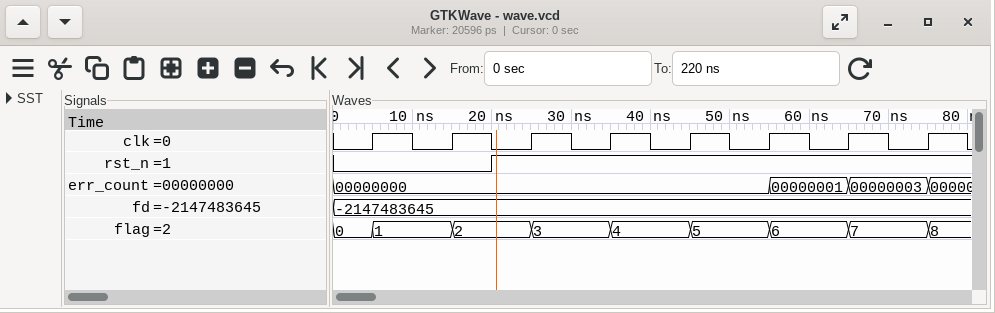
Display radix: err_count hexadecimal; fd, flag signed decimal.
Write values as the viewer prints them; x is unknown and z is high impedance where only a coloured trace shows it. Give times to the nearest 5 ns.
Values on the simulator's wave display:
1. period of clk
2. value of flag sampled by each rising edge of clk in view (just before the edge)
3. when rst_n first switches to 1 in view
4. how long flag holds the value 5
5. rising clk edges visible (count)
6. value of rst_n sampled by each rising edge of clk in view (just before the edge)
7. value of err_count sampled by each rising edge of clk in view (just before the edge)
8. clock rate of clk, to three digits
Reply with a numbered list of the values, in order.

1. 10 ns
2. 0, 1, 2, 3, 4, 5, 6, 7
3. 20 ns
4. 10 ns
5. 8
6. 0 0 1 1 1 1 1 1
7. 00000000, 00000000, 00000000, 00000000, 00000000, 00000000, 00000001, 00000003
8. 100 MHz
